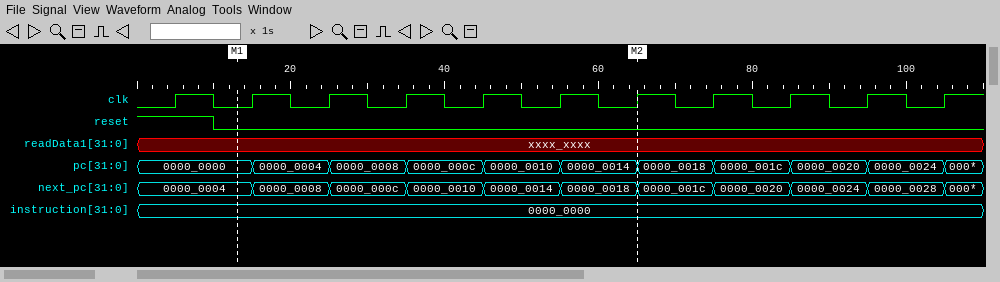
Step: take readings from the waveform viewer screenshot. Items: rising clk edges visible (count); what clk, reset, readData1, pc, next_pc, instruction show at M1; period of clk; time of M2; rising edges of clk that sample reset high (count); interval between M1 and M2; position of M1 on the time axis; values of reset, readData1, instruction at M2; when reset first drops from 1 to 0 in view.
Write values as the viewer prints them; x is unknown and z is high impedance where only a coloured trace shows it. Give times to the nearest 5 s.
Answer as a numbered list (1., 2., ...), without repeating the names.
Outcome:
1. 11
2. clk=0, reset=0, readData1=xxxx_xxxx, pc=0000_0000, next_pc=0000_0004, instruction=0000_0000
3. 10 s
4. 65 s
5. 1
6. 50 s
7. 15 s
8. reset=0, readData1=xxxx_xxxx, instruction=0000_0000
9. 10 s
